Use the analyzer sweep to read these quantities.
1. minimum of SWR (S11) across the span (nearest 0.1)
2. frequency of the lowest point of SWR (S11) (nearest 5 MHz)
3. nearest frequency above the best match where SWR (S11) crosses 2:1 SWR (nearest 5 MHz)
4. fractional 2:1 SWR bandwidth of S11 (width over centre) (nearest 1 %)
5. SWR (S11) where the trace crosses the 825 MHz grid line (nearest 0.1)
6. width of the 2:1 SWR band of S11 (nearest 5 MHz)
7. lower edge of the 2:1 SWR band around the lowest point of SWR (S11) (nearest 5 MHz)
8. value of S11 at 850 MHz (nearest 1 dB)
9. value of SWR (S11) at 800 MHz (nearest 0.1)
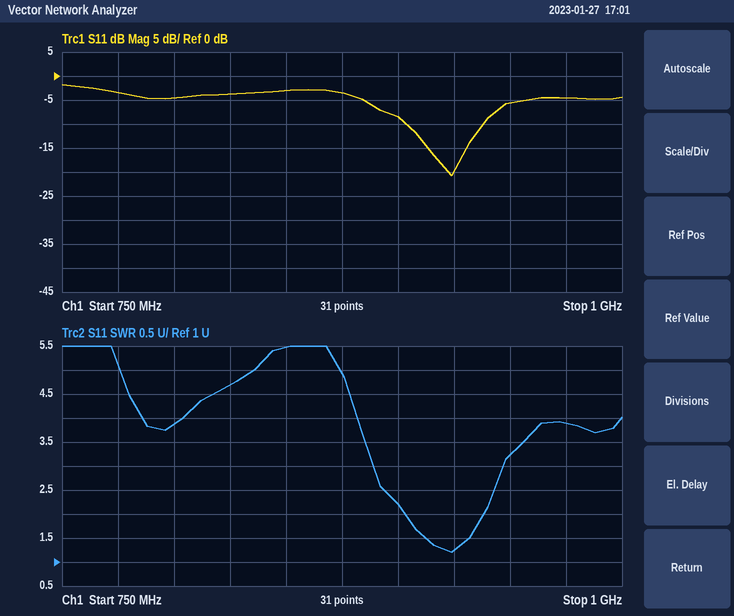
1.2
925 MHz
940 MHz
4 %
4.7
35 MHz
905 MHz
-3 dB
3.9
